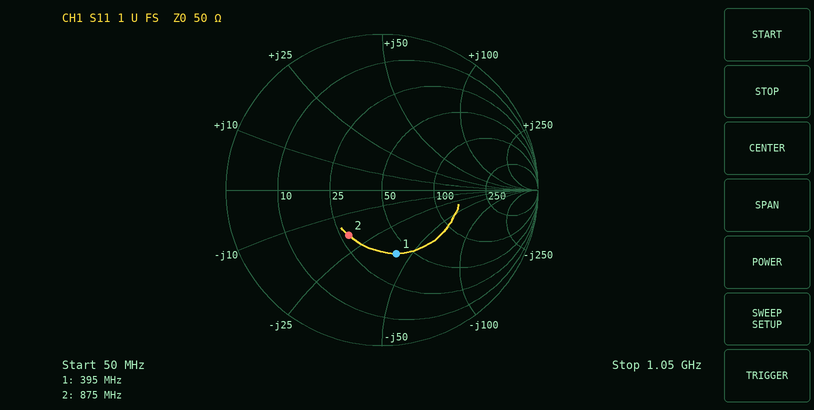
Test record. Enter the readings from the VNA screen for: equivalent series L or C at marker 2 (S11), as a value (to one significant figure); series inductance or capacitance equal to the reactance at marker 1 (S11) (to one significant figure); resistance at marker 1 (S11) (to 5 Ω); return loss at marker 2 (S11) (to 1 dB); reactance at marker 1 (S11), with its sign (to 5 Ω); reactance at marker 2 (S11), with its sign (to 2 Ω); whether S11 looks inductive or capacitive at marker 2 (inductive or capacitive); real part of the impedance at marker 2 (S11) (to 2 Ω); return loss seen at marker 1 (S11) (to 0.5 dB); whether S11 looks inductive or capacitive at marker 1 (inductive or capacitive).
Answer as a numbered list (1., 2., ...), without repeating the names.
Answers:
1. 10 pF
2. 10 pF
3. 40 Ω
4. 9 dB
5. -40 Ω
6. -18 Ω
7. capacitive
8. 28 Ω
9. 7.5 dB
10. capacitive
